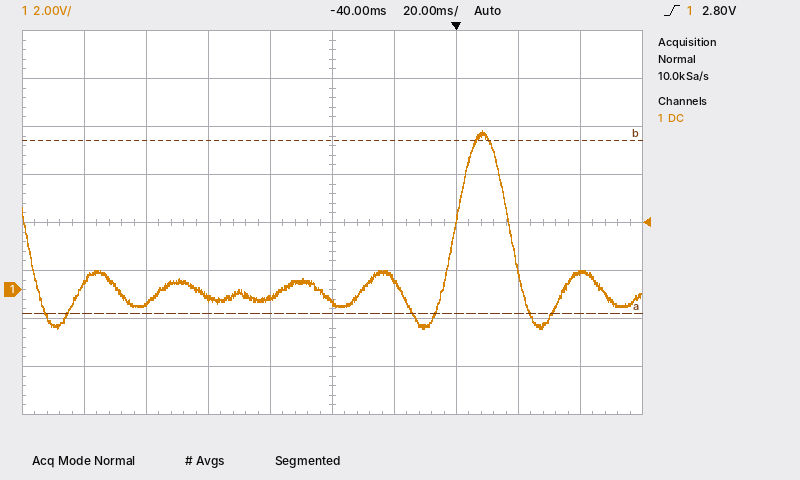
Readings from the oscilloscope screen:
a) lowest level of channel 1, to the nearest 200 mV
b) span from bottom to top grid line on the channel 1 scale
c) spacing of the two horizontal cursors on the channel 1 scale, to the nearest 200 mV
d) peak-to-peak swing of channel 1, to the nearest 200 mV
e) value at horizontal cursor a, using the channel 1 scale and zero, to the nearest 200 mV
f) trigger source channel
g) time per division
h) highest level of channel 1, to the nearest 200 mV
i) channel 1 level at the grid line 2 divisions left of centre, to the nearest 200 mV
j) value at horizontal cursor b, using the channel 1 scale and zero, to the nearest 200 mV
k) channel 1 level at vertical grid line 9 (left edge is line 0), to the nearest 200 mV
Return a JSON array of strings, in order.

["-1.6 V", "16 V", "7.2 V", "8.2 V", "-1.0 V", "channel 1", "20 ms", "6.6 V", "-400 mV", "6.2 V", "800 mV"]
